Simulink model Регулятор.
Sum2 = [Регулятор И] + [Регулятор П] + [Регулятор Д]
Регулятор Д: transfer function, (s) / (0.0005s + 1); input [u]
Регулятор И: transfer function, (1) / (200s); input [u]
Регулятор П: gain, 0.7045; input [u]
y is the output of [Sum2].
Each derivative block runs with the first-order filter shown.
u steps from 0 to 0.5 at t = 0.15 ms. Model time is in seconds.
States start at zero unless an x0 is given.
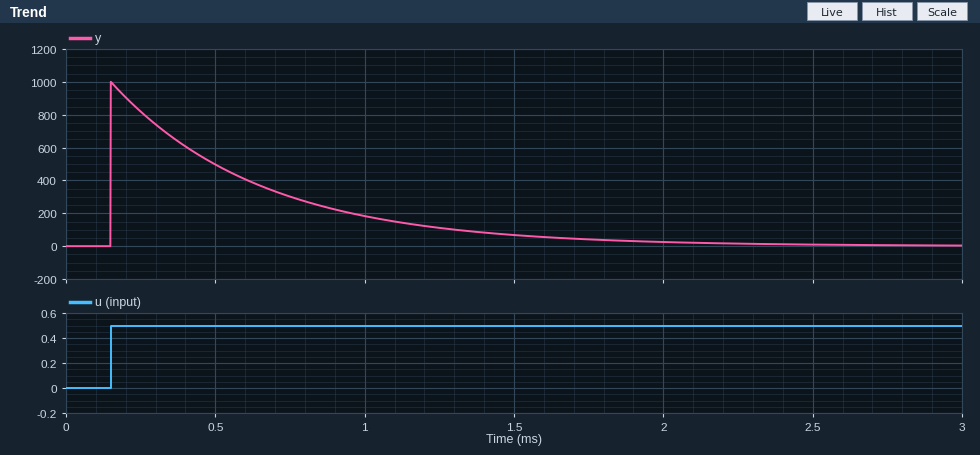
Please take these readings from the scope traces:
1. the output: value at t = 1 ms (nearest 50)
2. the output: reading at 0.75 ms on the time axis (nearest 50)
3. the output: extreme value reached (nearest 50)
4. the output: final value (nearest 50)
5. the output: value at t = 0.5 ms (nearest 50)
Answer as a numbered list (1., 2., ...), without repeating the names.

1. 200
2. 300
3. 1000
4. 0
5. 500
